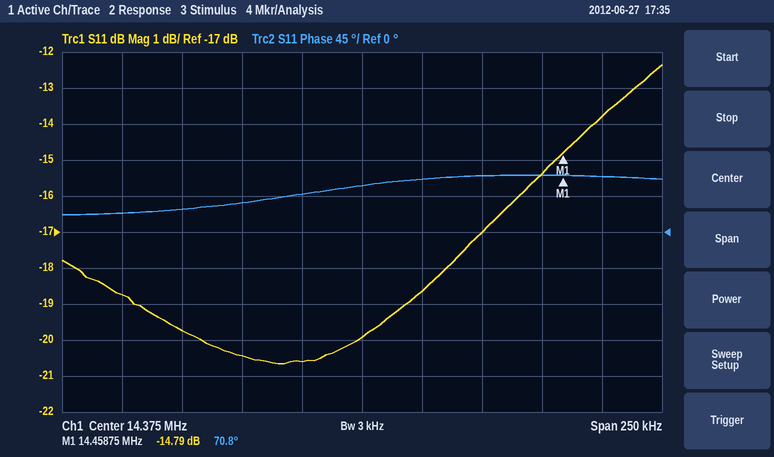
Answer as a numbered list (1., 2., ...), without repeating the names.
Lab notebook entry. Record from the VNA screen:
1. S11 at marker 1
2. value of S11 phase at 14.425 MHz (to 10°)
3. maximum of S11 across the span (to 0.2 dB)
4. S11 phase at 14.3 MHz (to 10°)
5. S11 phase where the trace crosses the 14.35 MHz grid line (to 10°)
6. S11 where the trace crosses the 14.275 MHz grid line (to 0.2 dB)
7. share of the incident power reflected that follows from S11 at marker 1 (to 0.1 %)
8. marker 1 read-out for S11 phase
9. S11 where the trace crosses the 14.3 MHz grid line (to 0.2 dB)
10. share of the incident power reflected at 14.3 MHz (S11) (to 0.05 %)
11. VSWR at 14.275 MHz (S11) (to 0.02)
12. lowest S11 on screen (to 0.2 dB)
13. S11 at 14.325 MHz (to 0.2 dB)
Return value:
1. -14.79 dB
2. 70°
3. -12.4 dB
4. 30°
5. 50°
6. -18.8 dB
7. 3.3 %
8. 70.8°
9. -19.8 dB
10. 1.05 %
11. 1.26
12. -20.6 dB
13. -20.4 dB
